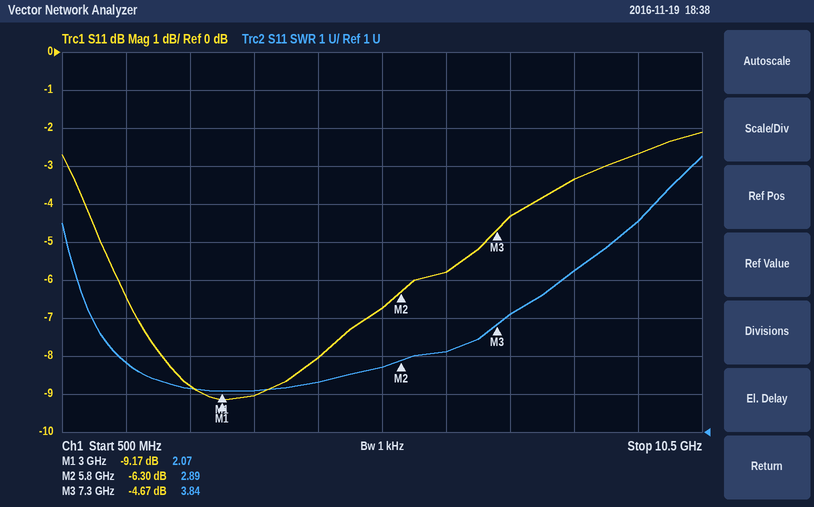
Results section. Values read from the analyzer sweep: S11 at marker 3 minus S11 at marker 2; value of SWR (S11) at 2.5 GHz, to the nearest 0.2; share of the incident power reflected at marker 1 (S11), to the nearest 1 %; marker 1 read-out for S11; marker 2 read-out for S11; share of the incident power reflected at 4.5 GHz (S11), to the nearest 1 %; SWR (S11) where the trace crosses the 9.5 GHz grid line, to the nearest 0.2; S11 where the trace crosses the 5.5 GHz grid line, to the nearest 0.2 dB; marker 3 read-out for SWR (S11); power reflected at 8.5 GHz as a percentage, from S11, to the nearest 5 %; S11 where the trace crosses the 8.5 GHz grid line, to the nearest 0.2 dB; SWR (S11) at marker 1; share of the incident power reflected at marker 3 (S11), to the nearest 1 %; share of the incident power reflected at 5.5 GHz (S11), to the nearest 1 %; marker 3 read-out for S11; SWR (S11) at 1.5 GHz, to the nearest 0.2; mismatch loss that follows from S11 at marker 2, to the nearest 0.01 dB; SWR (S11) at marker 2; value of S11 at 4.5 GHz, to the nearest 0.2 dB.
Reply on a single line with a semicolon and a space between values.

1.63 dB; 2.2; 12 %; -9.17 dB; -6.30 dB; 16 %; 6.6; -6.8 dB; 3.84; 45 %; -3.4 dB; 2.07; 34 %; 21 %; -4.67 dB; 2.8; 1.16 dB; 2.89; -8.0 dB
